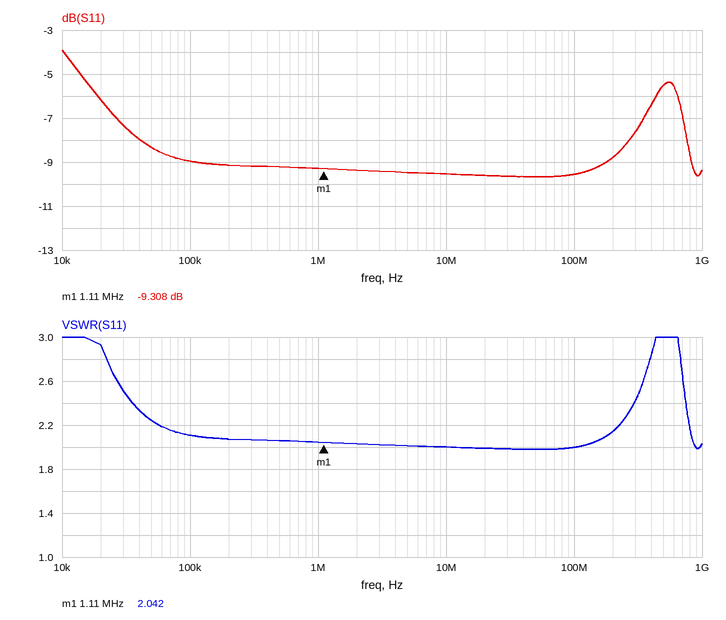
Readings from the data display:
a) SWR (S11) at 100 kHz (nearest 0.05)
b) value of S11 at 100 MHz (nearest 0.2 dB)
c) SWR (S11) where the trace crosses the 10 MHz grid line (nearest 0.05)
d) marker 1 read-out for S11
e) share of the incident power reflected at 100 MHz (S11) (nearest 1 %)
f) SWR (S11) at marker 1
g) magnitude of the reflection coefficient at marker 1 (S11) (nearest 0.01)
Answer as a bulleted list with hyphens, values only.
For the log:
- 2.10
- -9.6 dB
- 2.00
- -9.308 dB
- 11 %
- 2.042
- 0.34
